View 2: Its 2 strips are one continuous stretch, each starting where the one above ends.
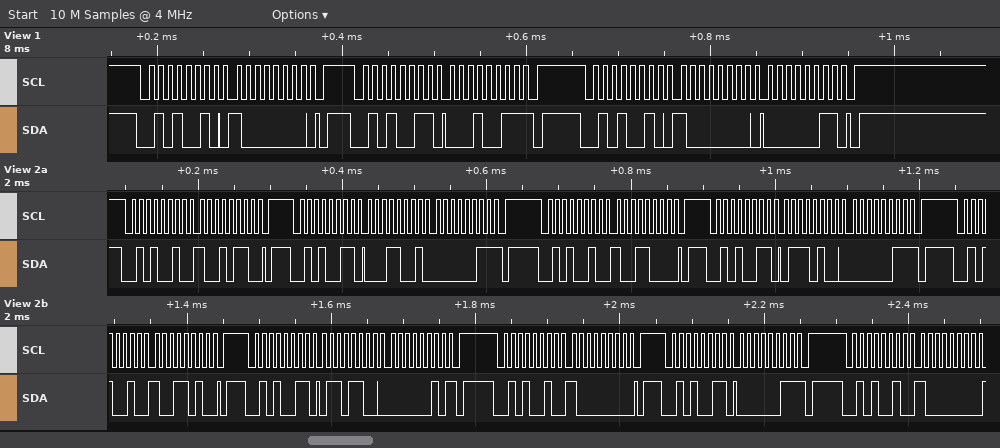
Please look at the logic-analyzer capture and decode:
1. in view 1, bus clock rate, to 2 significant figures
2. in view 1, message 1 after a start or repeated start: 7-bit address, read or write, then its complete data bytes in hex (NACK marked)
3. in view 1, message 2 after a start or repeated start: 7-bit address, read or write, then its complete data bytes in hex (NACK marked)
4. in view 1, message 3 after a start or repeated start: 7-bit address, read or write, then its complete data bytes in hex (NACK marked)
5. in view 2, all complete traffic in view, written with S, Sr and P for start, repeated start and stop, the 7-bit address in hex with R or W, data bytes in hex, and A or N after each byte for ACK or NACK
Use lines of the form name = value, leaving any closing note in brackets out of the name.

in view 1, bus clock rate, to 2 significant figures = 100 kHz
in view 1, message 1 after a start or repeated start: 7-bit address, read or write, then its complete data bytes in hex = 0x29 write: 80
in view 1, message 2 after a start or repeated start: 7-bit address, read or write, then its complete data bytes in hex = 0x29 read: 13 NACK
in view 1, message 3 after a start or repeated start: 7-bit address, read or write, then its complete data bytes in hex = 0x29 write: 80 03
in view 2, all complete traffic in view, written with S, Sr and P for start, repeated start and stop, the 7-bit address in hex with R or W, data bytes in hex, and A or N after each byte for ACK or NACK = S 29W A 96 A P S 29R A 19 A 03 N P S 29W A 98 A P S 29R A 74 A 03 N P S 29W A 9A A P S 29R A 6C A 02 N P S 29W A 80 A P S 29R A 03 N P S 29W A 80 A
